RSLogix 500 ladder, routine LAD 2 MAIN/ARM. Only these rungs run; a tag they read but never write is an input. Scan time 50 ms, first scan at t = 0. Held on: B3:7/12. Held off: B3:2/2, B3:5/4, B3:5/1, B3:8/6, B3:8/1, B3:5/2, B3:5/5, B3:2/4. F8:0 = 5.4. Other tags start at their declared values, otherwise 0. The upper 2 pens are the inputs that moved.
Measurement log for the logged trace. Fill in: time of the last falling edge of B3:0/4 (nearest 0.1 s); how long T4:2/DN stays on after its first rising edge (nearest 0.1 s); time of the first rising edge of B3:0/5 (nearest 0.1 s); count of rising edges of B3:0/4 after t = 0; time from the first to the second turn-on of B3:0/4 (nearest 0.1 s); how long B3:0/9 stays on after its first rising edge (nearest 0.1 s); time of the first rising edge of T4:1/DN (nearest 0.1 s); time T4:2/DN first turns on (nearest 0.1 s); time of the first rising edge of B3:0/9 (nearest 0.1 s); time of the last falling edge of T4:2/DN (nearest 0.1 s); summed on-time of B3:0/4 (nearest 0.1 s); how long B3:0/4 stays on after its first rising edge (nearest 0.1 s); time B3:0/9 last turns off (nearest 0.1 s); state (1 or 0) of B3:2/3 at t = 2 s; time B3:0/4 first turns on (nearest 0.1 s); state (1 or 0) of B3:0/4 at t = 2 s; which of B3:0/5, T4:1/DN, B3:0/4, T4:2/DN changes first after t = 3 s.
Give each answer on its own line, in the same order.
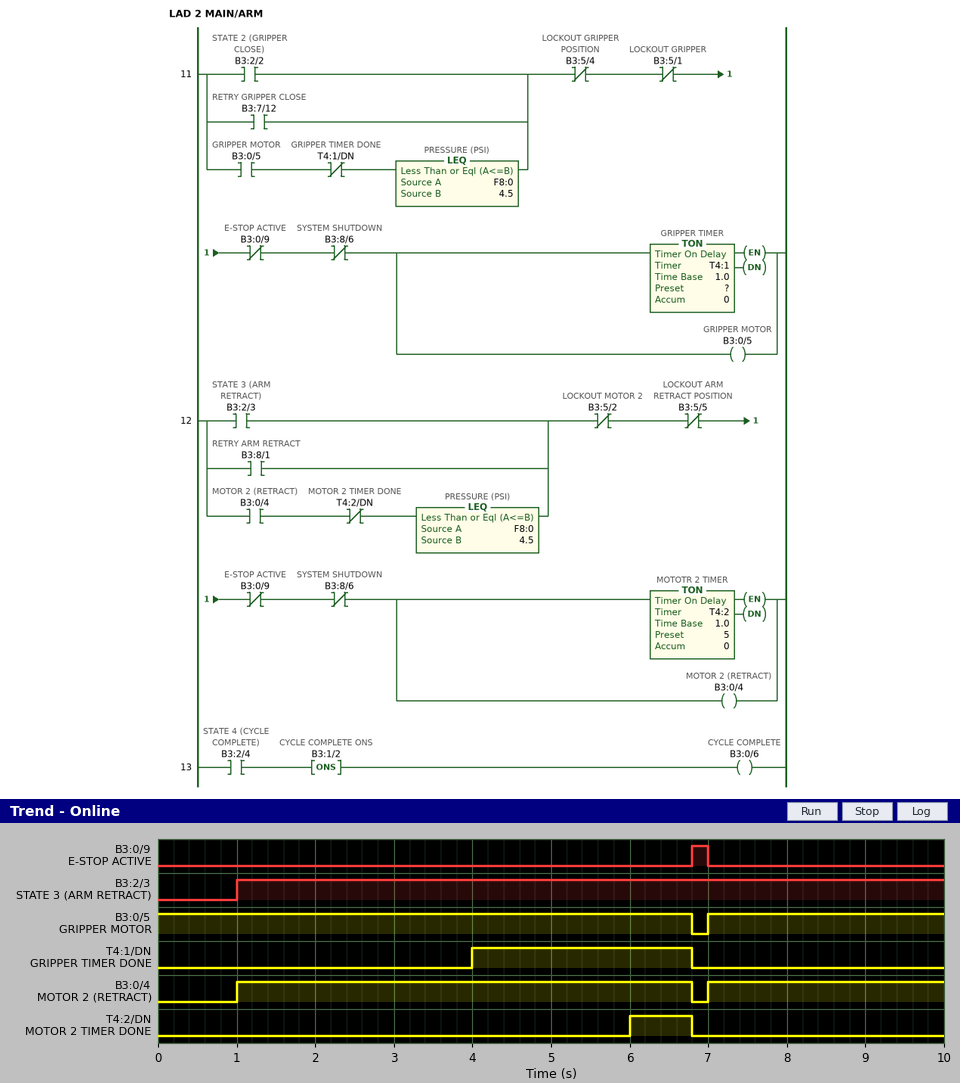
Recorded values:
6.8 s
0.8 s
7.0 s
2
6.0 s
0.2 s
4.0 s
6.0 s
6.8 s
6.8 s
8.8 s
5.8 s
7.0 s
1
1.0 s
1
T4:1/DN
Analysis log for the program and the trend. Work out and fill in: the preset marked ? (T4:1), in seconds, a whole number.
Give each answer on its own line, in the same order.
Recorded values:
4 s
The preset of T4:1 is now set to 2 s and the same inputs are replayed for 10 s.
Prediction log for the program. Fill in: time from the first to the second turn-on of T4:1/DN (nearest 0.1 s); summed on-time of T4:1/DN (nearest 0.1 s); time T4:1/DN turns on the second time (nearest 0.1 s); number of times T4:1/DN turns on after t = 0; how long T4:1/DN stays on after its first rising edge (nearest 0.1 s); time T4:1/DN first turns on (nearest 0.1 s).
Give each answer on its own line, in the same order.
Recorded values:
7.0 s
5.8 s
9.0 s
2
4.8 s
2.0 s
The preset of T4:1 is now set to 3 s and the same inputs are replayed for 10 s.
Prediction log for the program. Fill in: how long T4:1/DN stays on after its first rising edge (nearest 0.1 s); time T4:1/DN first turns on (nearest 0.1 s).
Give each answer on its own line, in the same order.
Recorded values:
3.8 s
3.0 s
